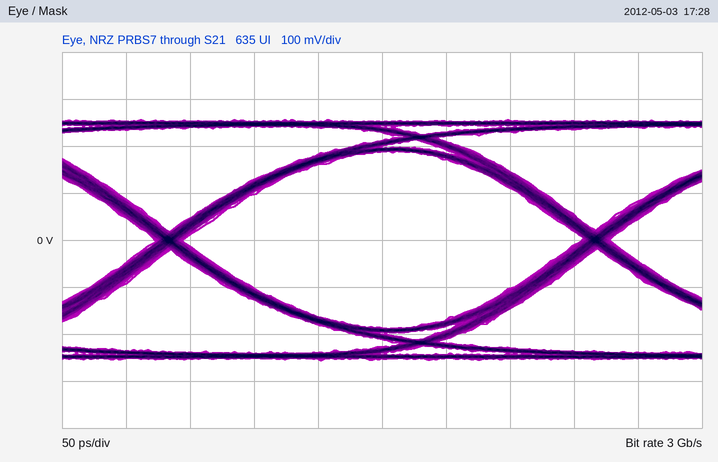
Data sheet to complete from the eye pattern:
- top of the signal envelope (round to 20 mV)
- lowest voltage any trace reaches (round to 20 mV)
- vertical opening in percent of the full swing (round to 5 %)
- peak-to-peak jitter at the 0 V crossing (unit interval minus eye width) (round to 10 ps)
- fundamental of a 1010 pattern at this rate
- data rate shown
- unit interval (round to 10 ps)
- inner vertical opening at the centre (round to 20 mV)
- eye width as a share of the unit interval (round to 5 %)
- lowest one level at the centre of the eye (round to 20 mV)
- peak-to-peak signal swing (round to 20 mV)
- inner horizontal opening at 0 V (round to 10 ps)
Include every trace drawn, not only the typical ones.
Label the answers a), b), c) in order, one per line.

a) 260 mV
b) -260 mV
c) 75 %
d) 20 ps
e) 1.5 GHz
f) 3 Gb/s
g) 330 ps
h) 380 mV
i) 95 %
j) 180 mV
k) 520 mV
l) 310 ps
